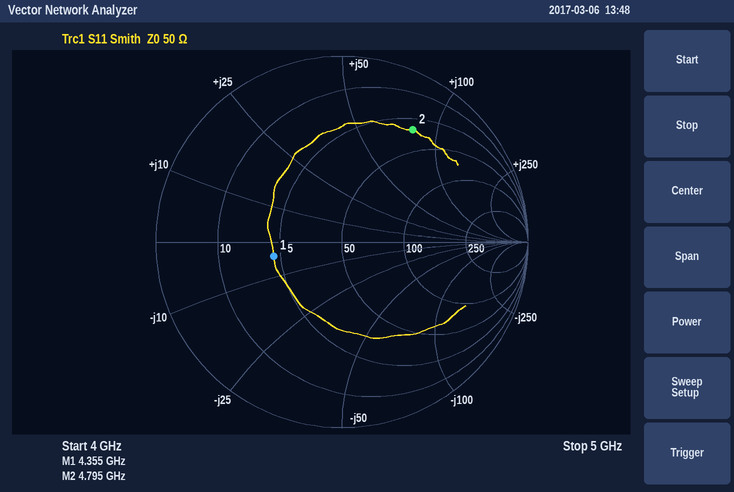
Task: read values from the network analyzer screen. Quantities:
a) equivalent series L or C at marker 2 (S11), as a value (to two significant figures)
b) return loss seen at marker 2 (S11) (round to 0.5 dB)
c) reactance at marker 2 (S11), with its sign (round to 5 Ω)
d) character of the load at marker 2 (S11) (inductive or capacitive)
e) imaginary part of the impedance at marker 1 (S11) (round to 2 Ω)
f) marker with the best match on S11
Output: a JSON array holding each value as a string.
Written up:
["2.7 nH", "3.0 dB", "+80 Ω", "inductive", "-4 Ω", "marker 1"]
